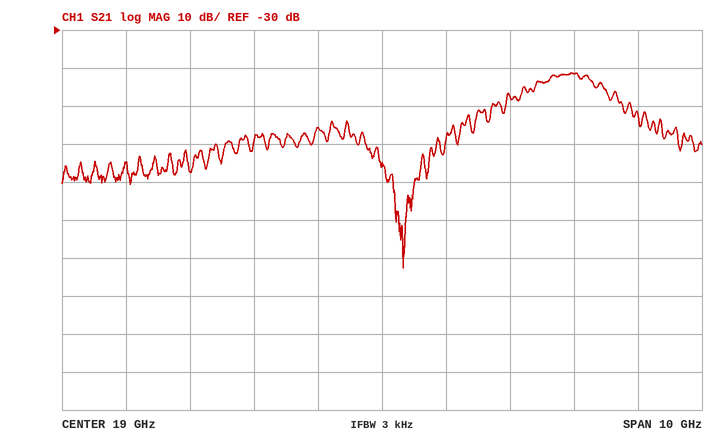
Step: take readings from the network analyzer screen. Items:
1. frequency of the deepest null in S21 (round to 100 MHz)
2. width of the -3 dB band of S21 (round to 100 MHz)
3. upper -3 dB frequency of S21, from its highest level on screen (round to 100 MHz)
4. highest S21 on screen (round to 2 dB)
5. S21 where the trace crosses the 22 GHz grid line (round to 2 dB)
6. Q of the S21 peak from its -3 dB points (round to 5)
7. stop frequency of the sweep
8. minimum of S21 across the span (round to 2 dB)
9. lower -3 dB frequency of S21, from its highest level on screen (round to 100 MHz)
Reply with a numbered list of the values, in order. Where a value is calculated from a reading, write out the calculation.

1. 19.3 GHz
2. 22.3 GHz − 21.4 GHz = 900 MHz
3. 22.3 GHz
4. -42 dB
5. -42 dB
6. 21.85 GHz / 900 MHz ≈ 24.3, so 25 to the nearest 5
7. 24 GHz
8. -92 dB
9. 21.4 GHz
